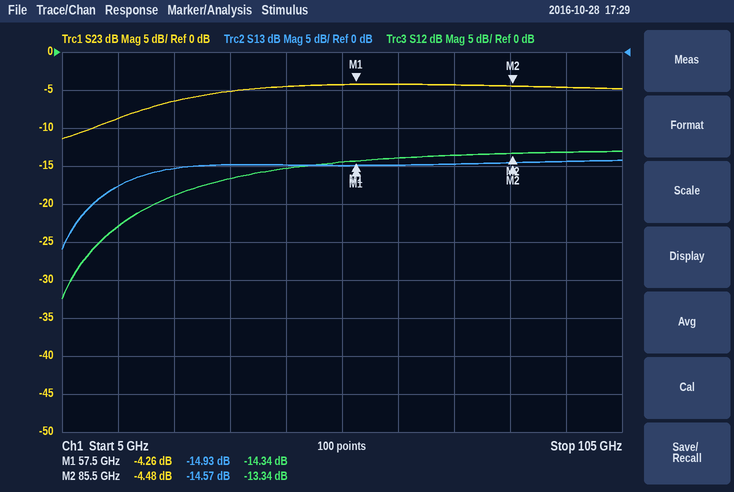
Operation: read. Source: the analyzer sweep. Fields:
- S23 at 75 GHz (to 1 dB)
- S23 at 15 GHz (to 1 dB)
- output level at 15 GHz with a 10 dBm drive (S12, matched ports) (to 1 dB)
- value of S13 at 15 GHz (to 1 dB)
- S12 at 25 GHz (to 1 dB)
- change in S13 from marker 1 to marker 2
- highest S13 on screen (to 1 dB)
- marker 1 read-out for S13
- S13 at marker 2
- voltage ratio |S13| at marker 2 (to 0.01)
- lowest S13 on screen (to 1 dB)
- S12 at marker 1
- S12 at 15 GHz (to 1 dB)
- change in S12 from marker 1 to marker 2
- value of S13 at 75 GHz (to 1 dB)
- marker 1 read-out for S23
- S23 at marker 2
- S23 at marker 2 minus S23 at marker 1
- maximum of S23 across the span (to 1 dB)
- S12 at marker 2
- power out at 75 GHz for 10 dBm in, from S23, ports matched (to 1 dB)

-4 dB
-9 dB
-13 dBm
-18 dB
-19 dB
0.36 dB
-14 dB
-14.93 dB
-14.57 dB
0.19
-26 dB
-14.34 dB
-23 dB
1.00 dB
-15 dB
-4.26 dB
-4.48 dB
-0.22 dB
-4 dB
-13.34 dB
6 dBm
